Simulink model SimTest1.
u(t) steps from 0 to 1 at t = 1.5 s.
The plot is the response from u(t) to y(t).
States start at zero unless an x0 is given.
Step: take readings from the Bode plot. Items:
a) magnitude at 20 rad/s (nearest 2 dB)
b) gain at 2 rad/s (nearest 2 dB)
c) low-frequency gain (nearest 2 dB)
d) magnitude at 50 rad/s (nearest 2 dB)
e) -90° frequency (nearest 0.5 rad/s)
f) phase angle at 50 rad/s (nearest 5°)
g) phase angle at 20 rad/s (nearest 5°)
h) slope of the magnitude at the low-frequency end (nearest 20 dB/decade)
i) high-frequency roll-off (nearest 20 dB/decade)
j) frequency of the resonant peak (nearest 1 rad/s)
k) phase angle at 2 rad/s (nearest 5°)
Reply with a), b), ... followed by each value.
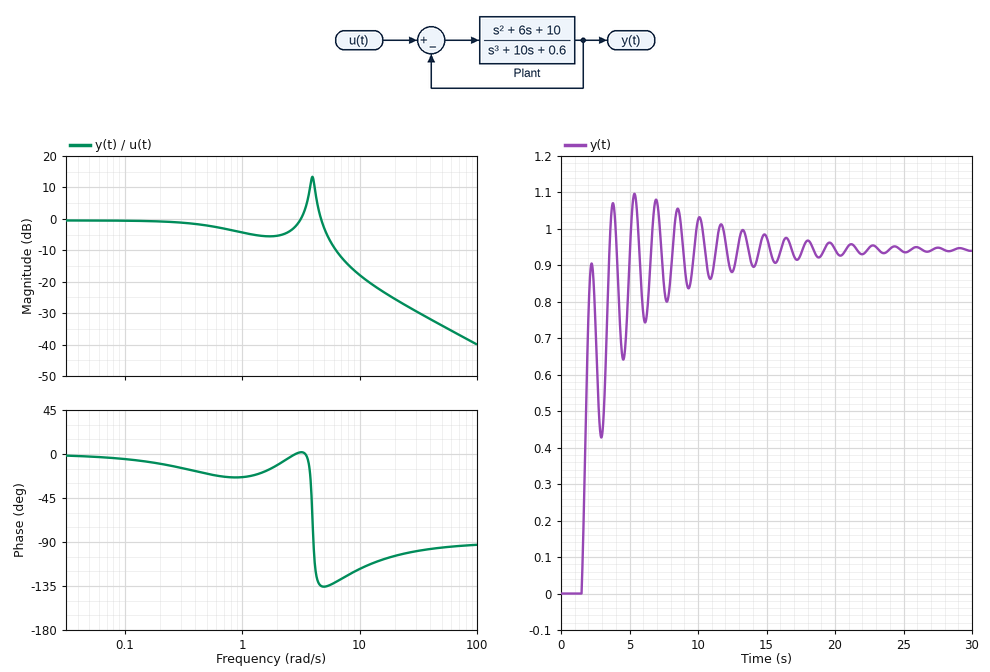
a) -26 dB
b) -6 dB
c) 0 dB
d) -34 dB
e) 4.0 rad/s
f) -95°
g) -105°
h) 0 dB/decade
i) -20 dB/decade
j) 4 rad/s
k) -10°
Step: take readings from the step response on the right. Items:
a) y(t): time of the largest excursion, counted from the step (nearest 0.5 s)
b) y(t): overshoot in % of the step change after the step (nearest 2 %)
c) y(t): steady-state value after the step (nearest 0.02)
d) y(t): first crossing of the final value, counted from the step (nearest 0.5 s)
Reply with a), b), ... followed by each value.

a) 4.0 s
b) 16 %
c) 0.94
d) 2.0 s
